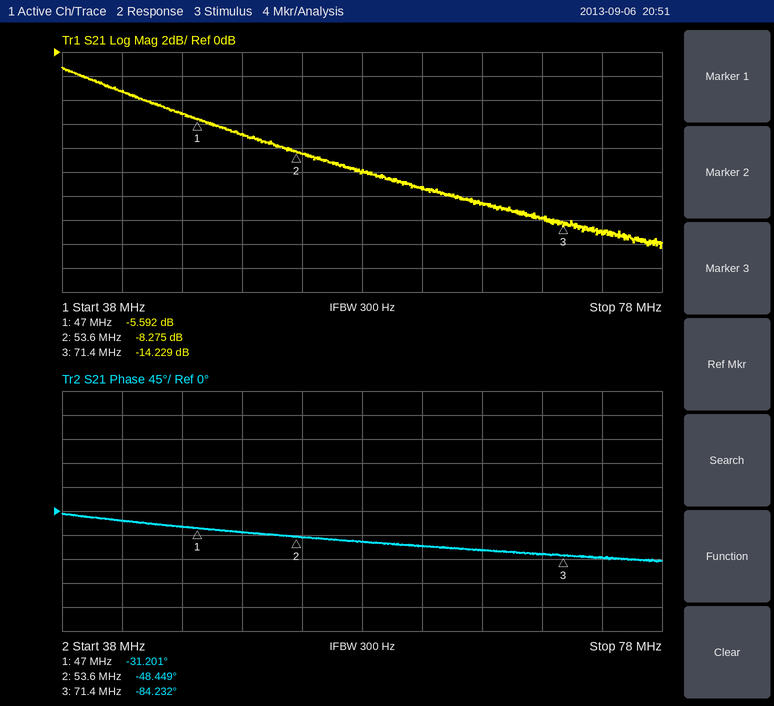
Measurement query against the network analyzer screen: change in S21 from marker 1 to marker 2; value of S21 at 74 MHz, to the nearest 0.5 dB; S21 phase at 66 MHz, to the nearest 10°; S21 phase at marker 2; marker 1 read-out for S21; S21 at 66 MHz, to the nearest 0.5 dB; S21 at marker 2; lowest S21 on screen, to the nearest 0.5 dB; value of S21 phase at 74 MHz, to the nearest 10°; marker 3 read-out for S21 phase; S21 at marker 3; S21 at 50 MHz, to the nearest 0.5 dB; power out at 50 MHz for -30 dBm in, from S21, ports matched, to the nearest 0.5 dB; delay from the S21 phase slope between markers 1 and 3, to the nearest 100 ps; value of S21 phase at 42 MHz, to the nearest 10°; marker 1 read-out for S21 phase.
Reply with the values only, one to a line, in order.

-2.683 dB
-15.0 dB
-70°
-48.449°
-5.592 dB
-12.5 dB
-8.275 dB
-16.5 dB
-90°
-84.232°
-14.229 dB
-7.0 dB
-37.0 dBm
6.0 ns
-20°
-31.201°
